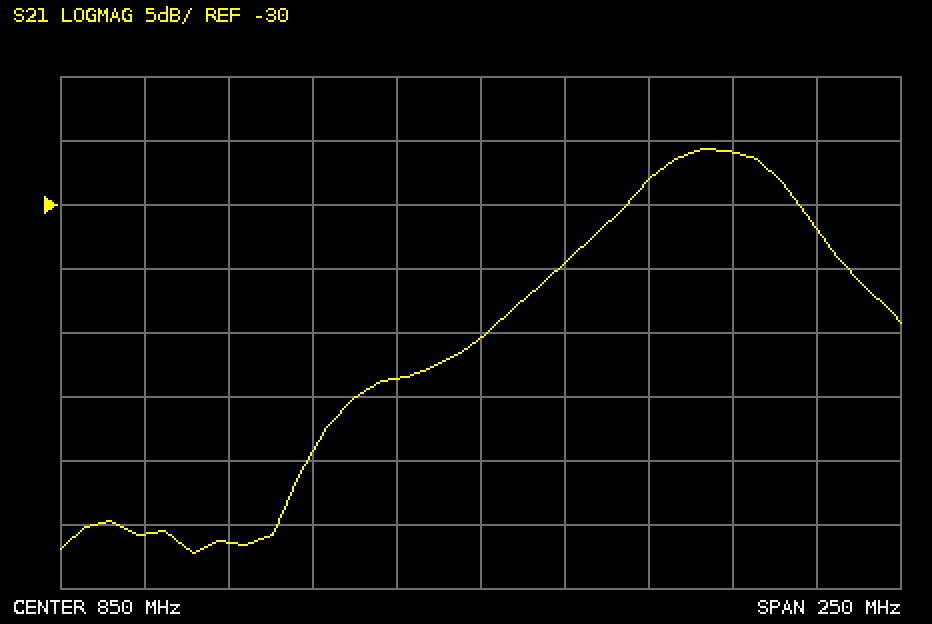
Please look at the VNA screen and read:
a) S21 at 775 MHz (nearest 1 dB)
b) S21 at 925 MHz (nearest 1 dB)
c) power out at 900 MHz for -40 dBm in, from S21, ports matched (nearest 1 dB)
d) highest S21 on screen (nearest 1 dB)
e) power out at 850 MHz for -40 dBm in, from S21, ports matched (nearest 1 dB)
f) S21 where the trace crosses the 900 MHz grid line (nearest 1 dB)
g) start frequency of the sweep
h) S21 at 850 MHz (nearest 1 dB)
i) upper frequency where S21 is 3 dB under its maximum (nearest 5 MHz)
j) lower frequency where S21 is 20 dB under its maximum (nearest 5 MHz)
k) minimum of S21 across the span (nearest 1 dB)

-56 dB
-26 dB
-68 dBm
-26 dB
-80 dBm
-28 dB
725 MHz
-40 dB
940 MHz
810 MHz
-57 dB
